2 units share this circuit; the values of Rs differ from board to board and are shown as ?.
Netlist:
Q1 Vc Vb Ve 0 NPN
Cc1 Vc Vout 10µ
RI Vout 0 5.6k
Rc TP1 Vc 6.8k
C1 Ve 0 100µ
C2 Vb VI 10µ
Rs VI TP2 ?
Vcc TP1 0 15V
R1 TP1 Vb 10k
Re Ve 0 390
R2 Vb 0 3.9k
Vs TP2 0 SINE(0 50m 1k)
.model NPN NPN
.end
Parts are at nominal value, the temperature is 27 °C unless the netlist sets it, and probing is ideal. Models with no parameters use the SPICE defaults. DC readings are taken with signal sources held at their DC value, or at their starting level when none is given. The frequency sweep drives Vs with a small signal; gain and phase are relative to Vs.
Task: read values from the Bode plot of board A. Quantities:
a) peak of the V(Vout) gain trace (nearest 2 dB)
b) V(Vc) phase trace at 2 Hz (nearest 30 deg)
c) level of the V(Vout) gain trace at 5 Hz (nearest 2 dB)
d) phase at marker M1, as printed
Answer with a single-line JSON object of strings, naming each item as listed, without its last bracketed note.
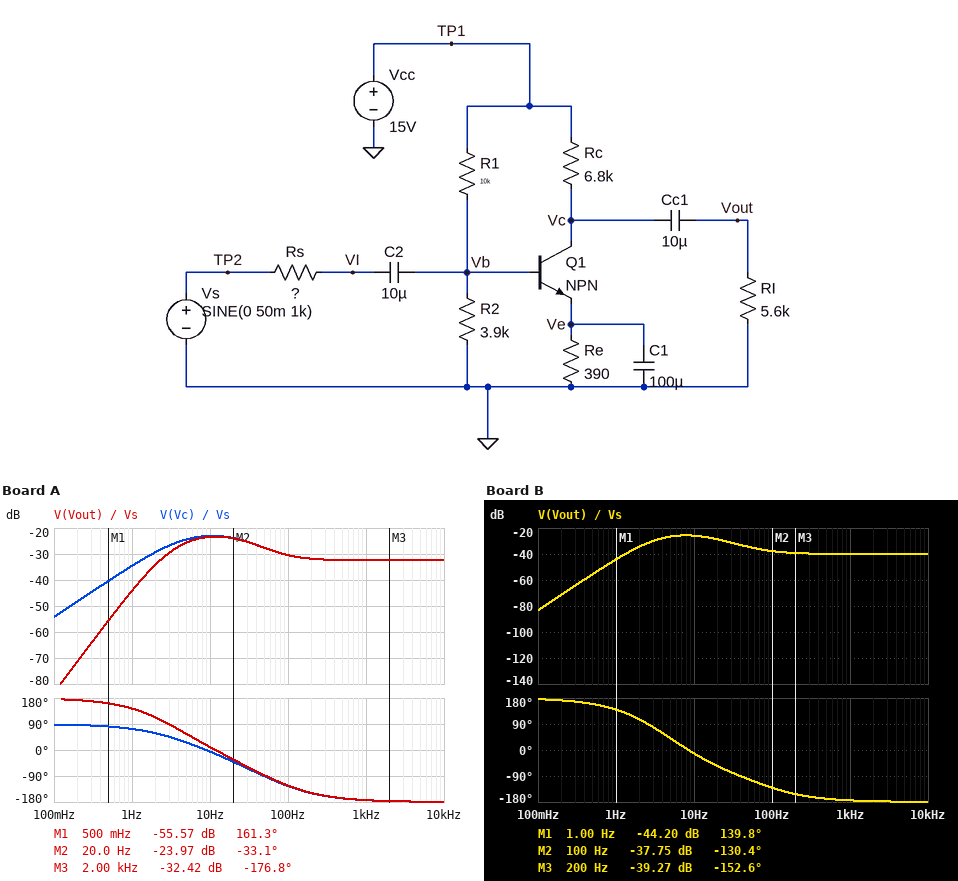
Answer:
{"peak of the V(Vout) gain trace": "-24 dB", "V(Vc) phase trace at 2 Hz": "60 deg", "level of the V(Vout) gain trace at 5 Hz": "-26 dB", "phase at marker M1, as printed": "161.3 deg"}
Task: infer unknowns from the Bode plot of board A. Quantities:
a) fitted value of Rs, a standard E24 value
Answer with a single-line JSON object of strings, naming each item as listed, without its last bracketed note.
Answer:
{"fitted value of Rs, a standard E24 value": "750 Ω"}
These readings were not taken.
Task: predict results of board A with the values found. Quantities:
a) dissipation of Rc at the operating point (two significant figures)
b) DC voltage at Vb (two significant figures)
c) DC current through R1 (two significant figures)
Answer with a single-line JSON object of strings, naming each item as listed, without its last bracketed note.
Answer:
{"dissipation of Rc at the operating point": "28 mW", "DC voltage at Vb": "1.9 V", "DC current through R1": "1.3 mA"}
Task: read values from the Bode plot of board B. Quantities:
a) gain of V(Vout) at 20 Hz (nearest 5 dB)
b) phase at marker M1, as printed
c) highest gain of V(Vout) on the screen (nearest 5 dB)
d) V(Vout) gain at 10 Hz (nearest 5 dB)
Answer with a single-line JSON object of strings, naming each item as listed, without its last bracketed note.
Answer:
{"gain of V(Vout) at 20 Hz": "-30 dB", "phase at marker M1, as printed": "139.8 deg", "highest gain of V(Vout) on the screen": "-25 dB", "V(Vout) gain at 10 Hz": "-25 dB"}
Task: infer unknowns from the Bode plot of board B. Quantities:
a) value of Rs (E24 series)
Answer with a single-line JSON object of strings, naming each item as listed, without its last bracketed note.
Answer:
{"value of Rs": "1.8 kΩ"}
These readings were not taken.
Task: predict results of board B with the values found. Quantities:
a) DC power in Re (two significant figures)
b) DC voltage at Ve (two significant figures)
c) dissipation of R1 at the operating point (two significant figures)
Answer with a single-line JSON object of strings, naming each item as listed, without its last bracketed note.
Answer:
{"DC power in Re": "3.2 mW", "DC voltage at Ve": "1.1 V", "dissipation of R1 at the operating point": "17 mW"}
